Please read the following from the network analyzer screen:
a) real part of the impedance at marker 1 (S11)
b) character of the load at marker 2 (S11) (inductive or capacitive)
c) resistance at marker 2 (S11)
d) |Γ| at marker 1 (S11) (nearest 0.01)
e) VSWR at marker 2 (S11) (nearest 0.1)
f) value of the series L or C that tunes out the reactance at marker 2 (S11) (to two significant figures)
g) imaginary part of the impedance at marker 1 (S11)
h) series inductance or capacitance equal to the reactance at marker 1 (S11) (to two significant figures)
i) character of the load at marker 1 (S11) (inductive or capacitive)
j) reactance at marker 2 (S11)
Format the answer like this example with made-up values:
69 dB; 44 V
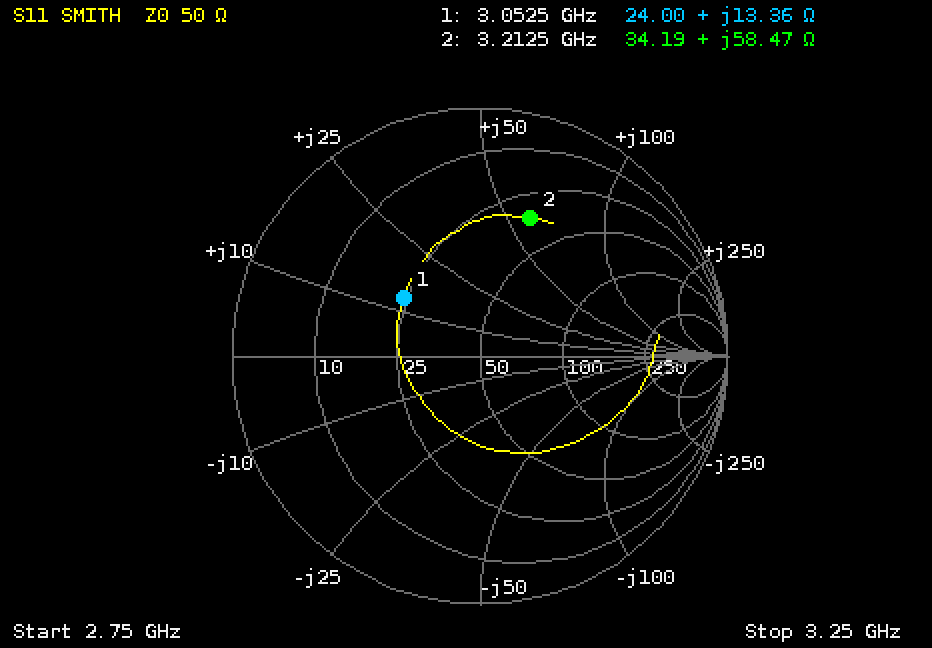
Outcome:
24.00 Ω; inductive; 34.19 Ω; 0.39; 3.9; 850 fF; +13.36 Ω; 700 pH; inductive; +58.47 Ω
